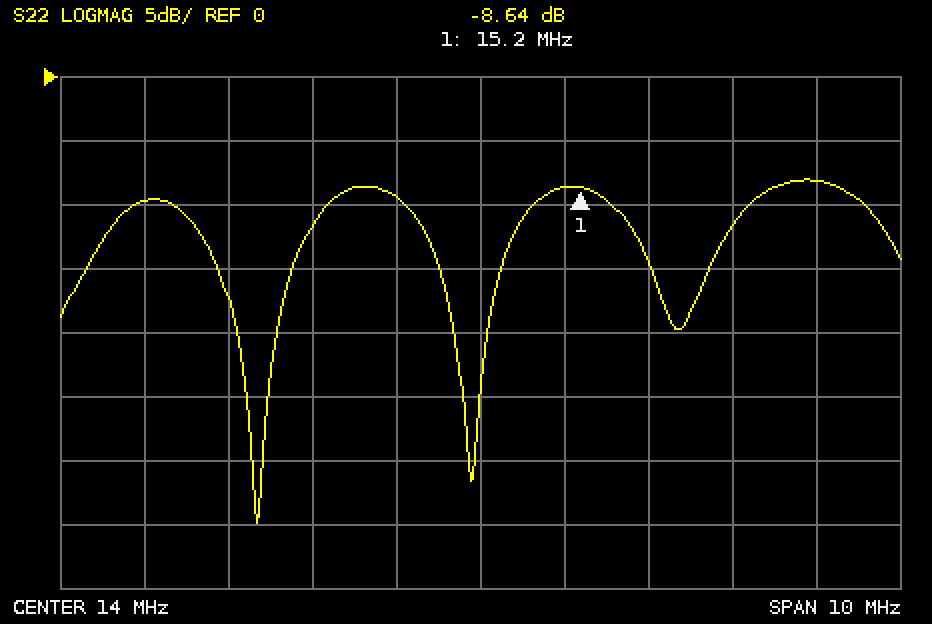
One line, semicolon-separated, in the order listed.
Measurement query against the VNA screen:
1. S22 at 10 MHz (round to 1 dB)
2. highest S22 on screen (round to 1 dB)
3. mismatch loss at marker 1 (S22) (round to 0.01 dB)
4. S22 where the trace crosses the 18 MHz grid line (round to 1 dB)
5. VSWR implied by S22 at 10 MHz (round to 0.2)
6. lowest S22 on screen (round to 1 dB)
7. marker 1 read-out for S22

-10 dB; -8 dB; 0.64 dB; -8 dB; 2.0; -35 dB; -8.64 dB
